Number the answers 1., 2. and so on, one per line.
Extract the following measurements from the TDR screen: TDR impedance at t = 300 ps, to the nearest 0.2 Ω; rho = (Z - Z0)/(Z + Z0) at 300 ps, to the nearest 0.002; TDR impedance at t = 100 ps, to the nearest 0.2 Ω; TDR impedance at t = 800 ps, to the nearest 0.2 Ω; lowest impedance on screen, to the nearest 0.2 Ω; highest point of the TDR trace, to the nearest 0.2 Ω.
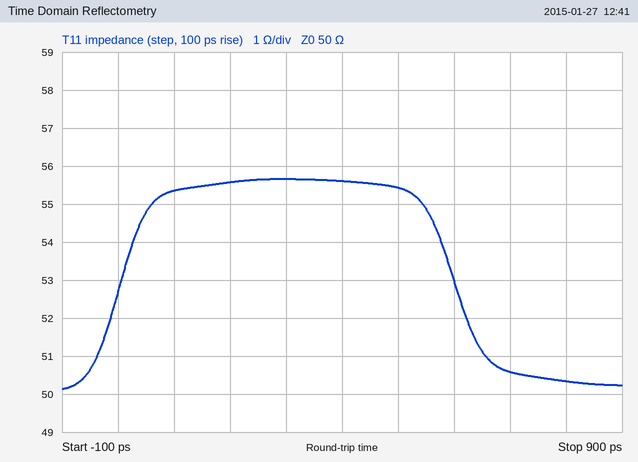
1. 55.6 Ω
2. +0.054
3. 55.4 Ω
4. 50.4 Ω
5. 50.2 Ω
6. 55.6 Ω
